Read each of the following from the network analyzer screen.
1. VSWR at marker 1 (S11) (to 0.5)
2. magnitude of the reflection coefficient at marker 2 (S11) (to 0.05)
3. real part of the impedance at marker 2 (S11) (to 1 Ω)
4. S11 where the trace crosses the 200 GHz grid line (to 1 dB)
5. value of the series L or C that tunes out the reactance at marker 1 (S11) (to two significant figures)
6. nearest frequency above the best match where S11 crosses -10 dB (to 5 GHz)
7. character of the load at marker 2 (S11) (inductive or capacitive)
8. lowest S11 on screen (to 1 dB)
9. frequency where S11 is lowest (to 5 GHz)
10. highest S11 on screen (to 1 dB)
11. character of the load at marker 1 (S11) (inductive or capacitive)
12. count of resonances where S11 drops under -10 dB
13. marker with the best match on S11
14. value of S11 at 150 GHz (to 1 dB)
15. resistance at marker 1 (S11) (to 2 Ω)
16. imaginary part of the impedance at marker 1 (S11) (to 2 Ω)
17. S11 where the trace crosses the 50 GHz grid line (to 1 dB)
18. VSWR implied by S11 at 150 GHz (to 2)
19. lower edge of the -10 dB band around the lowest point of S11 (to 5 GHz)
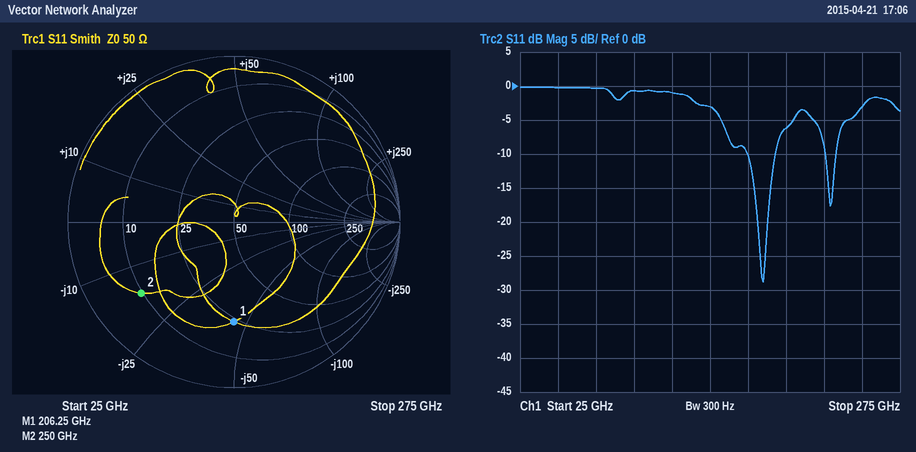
4.0
0.70
10 Ω
-6 dB
34 pH
195 GHz
capacitive
-29 dB
185 GHz
0 dB
capacitive
2
marker 1
-3 dB
24 Ω
-44 Ω
0 dB
6
175 GHz
